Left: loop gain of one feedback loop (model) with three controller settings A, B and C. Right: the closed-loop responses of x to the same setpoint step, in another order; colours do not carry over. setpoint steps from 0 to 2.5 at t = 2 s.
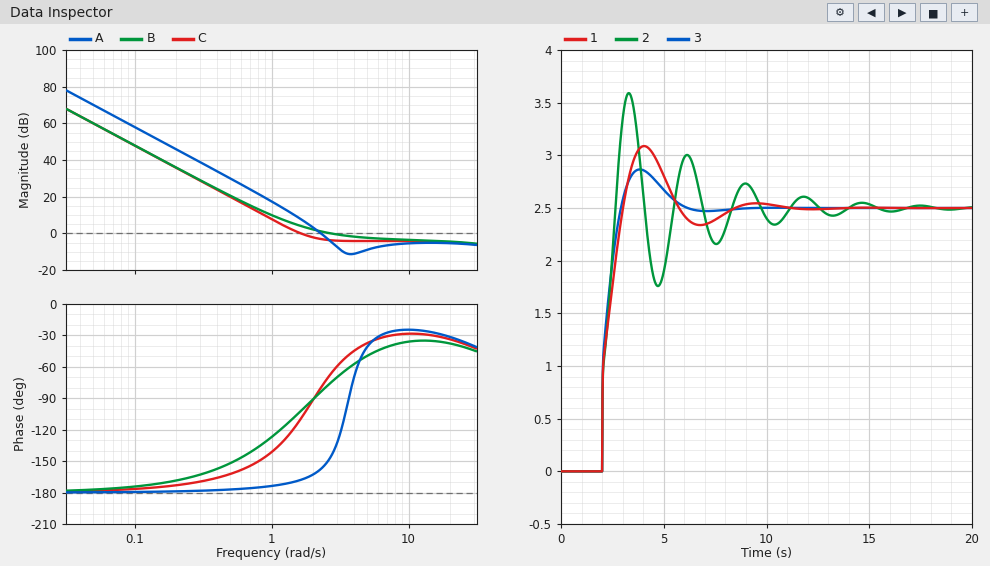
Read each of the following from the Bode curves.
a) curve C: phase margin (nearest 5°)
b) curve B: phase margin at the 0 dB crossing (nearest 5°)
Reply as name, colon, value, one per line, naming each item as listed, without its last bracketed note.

curve C: phase margin: 70°
curve B: phase margin at the 0 dB crossing: 105°
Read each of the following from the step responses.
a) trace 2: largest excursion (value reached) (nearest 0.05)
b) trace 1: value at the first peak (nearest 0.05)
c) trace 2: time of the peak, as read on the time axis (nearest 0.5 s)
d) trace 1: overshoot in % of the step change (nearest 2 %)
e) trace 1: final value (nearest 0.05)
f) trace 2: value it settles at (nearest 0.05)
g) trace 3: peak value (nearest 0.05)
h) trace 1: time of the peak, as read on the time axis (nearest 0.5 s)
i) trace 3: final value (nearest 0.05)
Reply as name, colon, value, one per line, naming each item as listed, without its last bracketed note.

trace 2: largest excursion (value reached): 3.60
trace 1: value at the first peak: 3.10
trace 2: time of the peak, as read on the time axis: 3.5 s
trace 1: overshoot in % of the step change: 24 %
trace 1: final value: 2.50
trace 2: value it settles at: 2.50
trace 3: peak value: 2.85
trace 1: time of the peak, as read on the time axis: 4.0 s
trace 3: final value: 2.50
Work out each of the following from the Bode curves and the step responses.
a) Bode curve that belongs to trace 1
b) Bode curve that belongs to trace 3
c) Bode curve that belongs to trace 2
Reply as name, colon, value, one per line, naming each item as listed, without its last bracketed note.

Bode curve that belongs to trace 1: C
Bode curve that belongs to trace 3: B
Bode curve that belongs to trace 2: A
